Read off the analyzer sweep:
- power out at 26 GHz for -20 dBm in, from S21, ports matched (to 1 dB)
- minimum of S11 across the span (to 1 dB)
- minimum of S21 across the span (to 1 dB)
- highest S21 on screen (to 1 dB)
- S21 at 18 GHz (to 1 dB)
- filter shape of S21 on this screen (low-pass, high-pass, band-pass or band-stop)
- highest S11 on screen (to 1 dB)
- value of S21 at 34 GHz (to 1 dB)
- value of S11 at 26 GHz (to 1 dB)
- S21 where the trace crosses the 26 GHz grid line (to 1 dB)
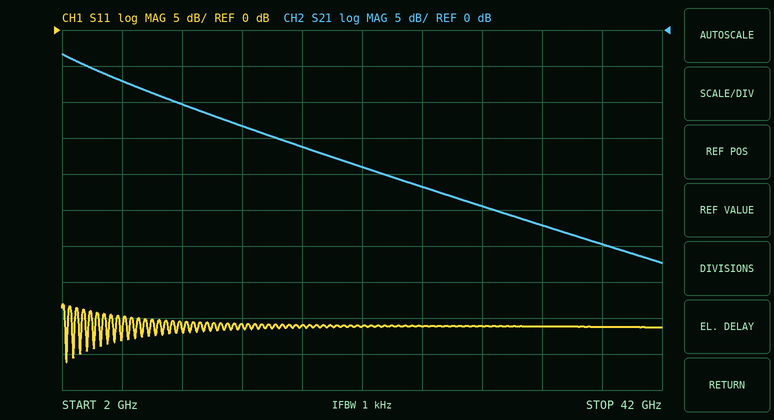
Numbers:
-42 dBm
-46 dB
-32 dB
-3 dB
-16 dB
low-pass
-38 dB
-27 dB
-41 dB
-22 dB
